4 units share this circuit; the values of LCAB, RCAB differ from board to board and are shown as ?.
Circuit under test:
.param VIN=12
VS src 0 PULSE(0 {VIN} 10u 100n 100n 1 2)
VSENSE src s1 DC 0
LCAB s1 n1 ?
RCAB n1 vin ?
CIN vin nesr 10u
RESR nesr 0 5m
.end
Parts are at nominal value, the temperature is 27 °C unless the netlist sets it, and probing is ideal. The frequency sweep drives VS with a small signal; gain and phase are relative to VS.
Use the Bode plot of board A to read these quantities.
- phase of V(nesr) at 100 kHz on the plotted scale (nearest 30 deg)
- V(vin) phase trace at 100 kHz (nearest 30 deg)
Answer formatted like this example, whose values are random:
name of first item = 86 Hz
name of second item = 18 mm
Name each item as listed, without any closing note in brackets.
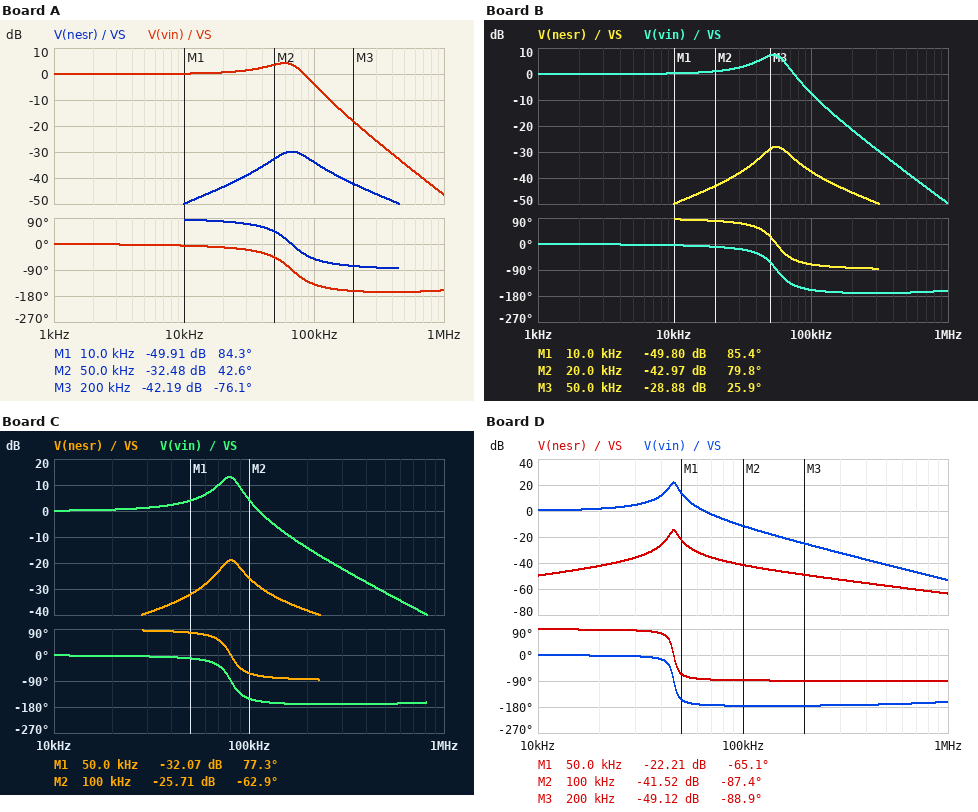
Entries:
phase of V(nesr) at 100 kHz on the plotted scale = -60 deg
V(vin) phase trace at 100 kHz = -150 deg
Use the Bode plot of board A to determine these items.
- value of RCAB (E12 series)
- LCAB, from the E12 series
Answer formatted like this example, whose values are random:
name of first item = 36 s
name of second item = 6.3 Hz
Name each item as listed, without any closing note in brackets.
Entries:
value of RCAB = 0.15 Ω
LCAB, from the E12 series = 560 nH
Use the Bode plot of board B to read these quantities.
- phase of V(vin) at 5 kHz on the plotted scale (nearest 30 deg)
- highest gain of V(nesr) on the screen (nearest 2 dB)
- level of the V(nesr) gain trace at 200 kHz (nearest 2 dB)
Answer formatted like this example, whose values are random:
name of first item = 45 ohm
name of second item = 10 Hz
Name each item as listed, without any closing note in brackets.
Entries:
phase of V(vin) at 5 kHz on the plotted scale = 0 deg
highest gain of V(nesr) on the screen = -28 dB
level of the V(nesr) gain trace at 200 kHz = -46 dB
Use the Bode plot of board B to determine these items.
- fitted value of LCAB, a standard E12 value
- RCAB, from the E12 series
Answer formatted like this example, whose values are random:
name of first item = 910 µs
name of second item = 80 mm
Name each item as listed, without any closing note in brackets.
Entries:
fitted value of LCAB, a standard E12 value = 820 nH
RCAB, from the E12 series = 0.12 Ω
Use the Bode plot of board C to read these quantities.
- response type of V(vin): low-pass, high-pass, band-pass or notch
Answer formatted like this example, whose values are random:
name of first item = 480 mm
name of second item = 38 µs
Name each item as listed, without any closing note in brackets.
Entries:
response type of V(vin): low-pass, high-pass, band-pass or notch = low-pass
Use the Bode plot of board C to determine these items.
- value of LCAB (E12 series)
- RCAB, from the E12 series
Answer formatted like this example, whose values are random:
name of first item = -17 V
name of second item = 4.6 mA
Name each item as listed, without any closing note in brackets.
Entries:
value of LCAB = 390 nH
RCAB, from the E12 series = 0.039 Ω
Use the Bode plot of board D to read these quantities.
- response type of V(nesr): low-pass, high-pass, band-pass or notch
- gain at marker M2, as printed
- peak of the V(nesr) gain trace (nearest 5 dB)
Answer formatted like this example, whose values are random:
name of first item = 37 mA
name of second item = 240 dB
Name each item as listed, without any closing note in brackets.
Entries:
response type of V(nesr): low-pass, high-pass, band-pass or notch = band-pass
gain at marker M2, as printed = -41.52 dB
peak of the V(nesr) gain trace = -15 dB
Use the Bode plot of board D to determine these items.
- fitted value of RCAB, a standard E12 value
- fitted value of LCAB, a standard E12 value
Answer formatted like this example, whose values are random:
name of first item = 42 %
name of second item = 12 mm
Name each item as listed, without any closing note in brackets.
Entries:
fitted value of RCAB, a standard E12 value = 0.022 Ω
fitted value of LCAB, a standard E12 value = 1.2 µH
